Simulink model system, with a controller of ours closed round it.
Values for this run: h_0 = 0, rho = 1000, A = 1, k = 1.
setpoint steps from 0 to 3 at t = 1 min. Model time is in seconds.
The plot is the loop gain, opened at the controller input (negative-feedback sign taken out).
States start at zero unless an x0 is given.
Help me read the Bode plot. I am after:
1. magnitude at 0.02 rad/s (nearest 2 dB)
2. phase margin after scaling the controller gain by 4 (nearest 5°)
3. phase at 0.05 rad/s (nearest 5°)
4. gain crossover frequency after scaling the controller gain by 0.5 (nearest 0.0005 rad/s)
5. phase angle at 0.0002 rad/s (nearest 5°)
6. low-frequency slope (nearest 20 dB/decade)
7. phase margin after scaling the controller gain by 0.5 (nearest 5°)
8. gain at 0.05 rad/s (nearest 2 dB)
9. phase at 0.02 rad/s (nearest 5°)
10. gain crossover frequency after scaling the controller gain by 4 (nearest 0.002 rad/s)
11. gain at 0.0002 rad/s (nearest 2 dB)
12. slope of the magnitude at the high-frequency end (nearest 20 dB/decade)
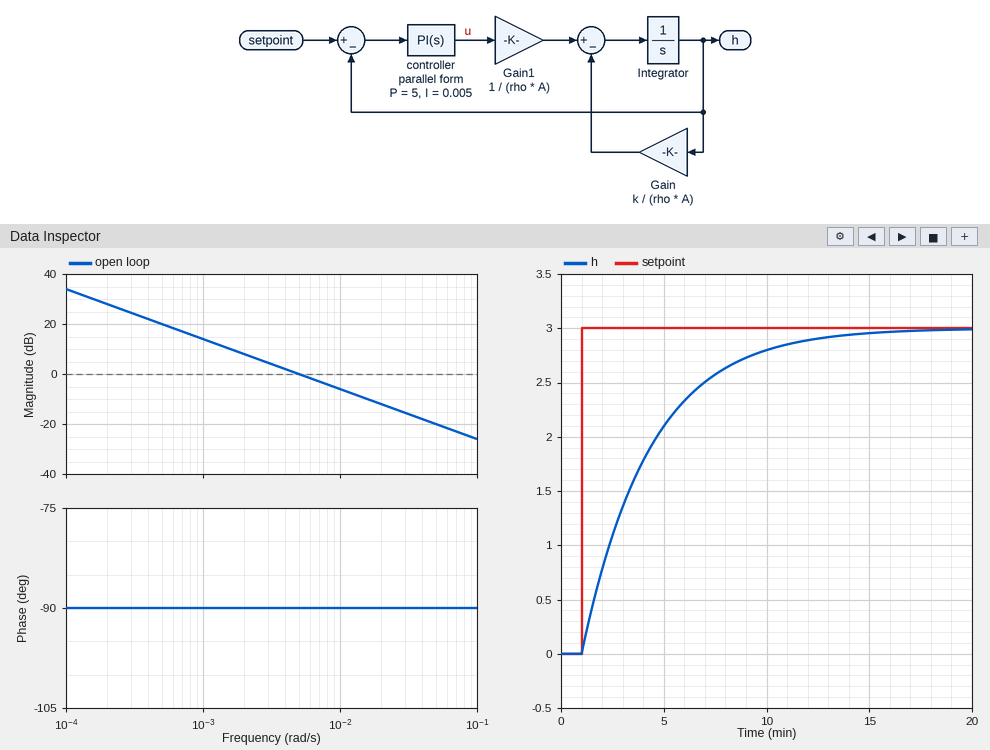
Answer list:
-12 dB
90°
-90°
0.0025 rad/s
-90°
-20 dB/decade
90°
-20 dB
-90°
0.020 rad/s
28 dB
-20 dB/decade
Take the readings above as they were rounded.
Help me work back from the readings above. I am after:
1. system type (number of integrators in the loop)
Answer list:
1
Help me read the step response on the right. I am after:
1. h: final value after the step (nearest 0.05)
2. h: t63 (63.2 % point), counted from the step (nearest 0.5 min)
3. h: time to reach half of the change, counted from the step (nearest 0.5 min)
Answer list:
3.00
3.5 min
2.5 min
